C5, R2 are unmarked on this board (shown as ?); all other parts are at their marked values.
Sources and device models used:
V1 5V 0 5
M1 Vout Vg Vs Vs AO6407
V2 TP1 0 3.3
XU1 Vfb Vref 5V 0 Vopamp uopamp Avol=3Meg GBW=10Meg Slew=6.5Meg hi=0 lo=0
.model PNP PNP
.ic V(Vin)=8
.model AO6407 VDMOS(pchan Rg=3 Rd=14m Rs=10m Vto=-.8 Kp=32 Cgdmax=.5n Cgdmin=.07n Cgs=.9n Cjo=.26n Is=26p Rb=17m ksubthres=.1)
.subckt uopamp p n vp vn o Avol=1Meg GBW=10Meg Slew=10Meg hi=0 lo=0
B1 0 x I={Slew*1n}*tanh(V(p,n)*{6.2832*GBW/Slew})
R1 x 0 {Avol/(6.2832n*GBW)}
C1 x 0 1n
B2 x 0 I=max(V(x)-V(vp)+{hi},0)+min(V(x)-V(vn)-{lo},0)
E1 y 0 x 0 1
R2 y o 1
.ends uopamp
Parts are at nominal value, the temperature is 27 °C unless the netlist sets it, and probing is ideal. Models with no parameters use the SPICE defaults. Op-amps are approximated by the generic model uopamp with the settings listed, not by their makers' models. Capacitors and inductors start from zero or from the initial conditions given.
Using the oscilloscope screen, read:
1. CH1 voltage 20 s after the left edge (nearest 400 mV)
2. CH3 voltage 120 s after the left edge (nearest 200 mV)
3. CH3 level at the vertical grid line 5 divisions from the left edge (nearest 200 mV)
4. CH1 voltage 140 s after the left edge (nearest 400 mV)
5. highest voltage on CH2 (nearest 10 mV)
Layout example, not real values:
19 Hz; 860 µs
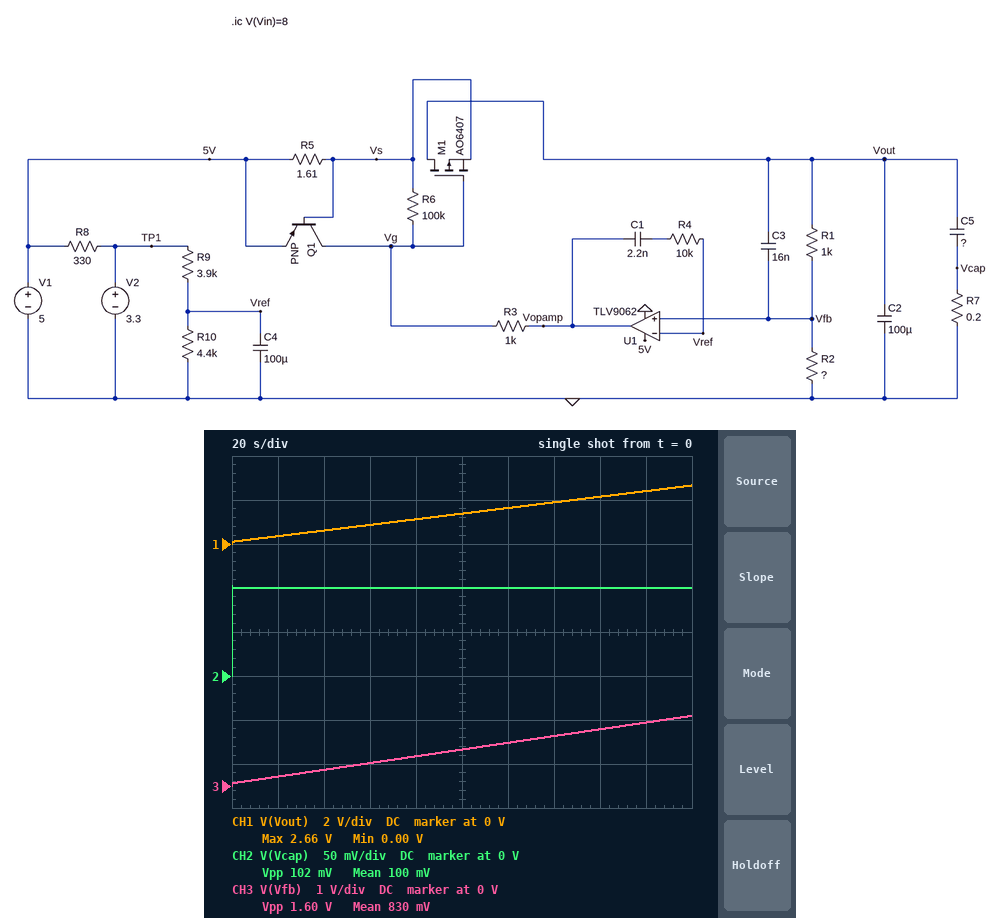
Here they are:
400 mV; 1.0 V; 800 mV; 2.0 V; 100 mV
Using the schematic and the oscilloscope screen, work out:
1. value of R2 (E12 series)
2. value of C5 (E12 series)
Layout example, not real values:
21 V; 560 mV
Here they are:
1.5 kΩ; 39 F
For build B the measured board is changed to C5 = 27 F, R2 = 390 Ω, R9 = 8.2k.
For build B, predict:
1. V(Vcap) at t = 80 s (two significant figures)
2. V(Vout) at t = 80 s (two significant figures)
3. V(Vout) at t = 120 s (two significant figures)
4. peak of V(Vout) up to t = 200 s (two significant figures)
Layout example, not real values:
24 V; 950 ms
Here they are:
100 mV; 1.6 V; 2.3 V; 3.8 V
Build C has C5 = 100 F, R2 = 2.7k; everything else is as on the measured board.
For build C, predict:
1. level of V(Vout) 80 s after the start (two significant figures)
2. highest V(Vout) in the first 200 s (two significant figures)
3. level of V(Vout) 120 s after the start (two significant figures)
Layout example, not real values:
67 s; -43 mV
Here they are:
500 mV; 1.1 V; 700 mV
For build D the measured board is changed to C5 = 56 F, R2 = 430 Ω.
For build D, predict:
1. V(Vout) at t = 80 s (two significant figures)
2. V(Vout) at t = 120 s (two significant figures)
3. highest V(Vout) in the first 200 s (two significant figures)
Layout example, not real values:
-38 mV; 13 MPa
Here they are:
810 mV; 1.2 V; 1.9 V
